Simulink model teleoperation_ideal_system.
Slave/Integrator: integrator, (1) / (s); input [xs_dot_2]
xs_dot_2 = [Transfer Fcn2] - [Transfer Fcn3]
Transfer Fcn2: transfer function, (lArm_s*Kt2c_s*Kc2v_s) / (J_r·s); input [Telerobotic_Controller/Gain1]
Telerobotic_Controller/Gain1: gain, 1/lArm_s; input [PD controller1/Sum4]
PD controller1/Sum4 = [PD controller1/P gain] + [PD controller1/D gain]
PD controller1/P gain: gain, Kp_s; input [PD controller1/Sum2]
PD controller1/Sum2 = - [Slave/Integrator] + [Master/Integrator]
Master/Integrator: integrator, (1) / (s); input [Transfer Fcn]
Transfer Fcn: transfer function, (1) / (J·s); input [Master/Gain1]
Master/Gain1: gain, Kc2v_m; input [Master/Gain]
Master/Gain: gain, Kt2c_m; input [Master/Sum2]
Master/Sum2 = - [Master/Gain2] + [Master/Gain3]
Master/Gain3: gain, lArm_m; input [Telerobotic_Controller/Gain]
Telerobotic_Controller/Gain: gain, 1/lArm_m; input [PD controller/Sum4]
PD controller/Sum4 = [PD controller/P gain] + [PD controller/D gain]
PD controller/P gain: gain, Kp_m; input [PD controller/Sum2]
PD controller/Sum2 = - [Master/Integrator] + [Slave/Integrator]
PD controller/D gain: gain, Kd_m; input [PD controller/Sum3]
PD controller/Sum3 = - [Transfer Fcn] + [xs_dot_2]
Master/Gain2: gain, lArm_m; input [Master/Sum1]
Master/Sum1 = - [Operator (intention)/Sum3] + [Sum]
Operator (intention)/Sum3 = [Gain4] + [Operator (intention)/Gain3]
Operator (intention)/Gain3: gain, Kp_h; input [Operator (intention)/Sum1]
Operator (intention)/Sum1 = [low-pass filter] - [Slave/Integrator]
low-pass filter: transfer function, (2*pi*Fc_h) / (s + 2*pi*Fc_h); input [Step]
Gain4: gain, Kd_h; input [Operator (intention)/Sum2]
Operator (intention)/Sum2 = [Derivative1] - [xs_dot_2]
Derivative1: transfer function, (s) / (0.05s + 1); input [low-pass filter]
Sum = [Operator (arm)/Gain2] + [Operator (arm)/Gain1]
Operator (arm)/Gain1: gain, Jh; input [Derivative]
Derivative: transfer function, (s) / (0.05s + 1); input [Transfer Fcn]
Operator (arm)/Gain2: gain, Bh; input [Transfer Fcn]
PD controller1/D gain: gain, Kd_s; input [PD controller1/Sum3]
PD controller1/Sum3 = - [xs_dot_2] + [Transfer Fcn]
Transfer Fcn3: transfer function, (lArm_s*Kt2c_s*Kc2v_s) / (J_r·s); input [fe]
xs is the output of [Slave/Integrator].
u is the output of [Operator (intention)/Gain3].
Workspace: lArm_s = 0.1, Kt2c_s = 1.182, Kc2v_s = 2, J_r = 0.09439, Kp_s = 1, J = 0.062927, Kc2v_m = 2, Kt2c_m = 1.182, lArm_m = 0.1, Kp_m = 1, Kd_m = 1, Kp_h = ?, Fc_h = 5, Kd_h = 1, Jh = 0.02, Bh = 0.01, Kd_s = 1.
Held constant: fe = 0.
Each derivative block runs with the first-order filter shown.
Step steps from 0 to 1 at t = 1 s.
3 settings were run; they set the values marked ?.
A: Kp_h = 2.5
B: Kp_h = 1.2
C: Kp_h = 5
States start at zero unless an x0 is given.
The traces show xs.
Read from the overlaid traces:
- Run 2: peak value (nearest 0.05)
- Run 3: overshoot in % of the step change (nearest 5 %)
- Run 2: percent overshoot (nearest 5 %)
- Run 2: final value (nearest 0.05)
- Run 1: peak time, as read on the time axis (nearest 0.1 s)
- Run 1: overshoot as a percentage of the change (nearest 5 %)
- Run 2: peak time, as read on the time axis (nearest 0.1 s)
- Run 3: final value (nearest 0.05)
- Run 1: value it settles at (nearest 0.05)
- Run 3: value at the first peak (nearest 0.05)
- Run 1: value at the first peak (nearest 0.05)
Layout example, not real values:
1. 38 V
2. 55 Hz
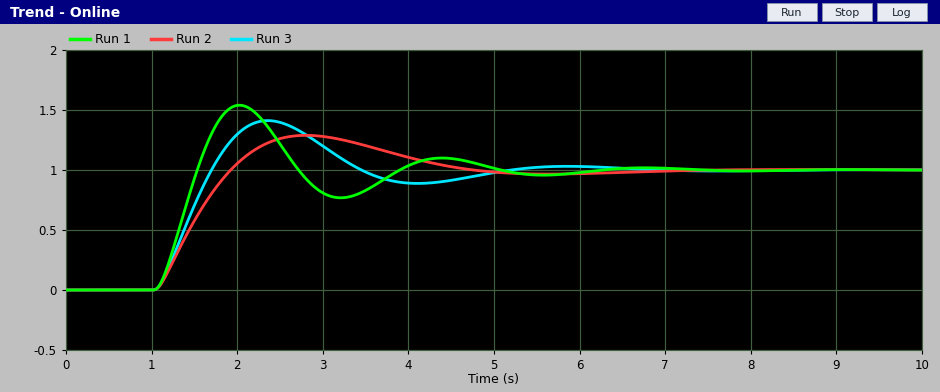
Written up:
1. 1.30
2. 40 %
3. 30 %
4. 1.00
5. 2.0 s
6. 55 %
7. 2.8 s
8. 1.00
9. 1.00
10. 1.40
11. 1.55
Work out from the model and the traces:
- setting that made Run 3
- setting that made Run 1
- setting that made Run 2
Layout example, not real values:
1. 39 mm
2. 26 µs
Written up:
1. A
2. C
3. B
